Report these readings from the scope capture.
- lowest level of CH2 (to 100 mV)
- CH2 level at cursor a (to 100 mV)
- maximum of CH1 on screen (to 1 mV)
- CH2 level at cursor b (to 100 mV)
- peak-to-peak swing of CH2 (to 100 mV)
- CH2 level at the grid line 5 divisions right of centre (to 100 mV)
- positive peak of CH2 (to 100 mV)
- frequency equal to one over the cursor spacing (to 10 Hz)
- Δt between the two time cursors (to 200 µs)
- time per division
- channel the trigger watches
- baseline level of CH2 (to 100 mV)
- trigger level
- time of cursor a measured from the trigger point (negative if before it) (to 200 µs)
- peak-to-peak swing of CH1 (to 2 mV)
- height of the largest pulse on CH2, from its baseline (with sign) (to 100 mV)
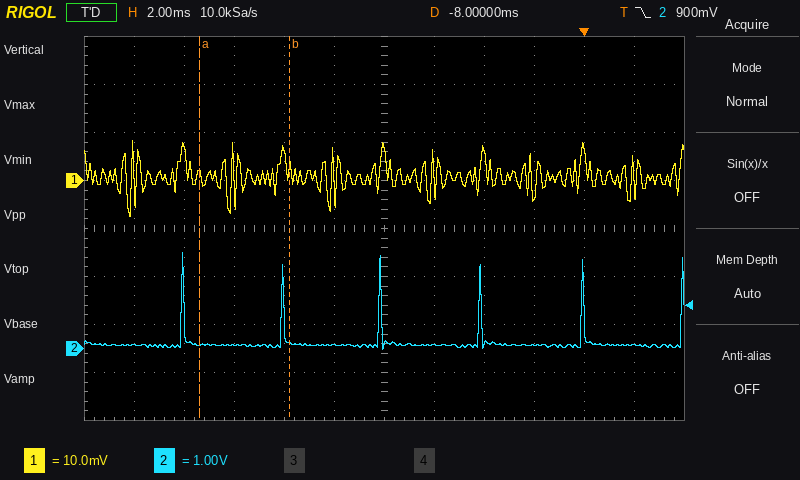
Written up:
0.0 V
100 mV
8 mV
100 mV
2.0 V
100 mV
2.0 V
280 Hz
3.6 ms
2 ms
CH2
100 mV
900 mV
-15.4 ms
16 mV
+1.9 V
